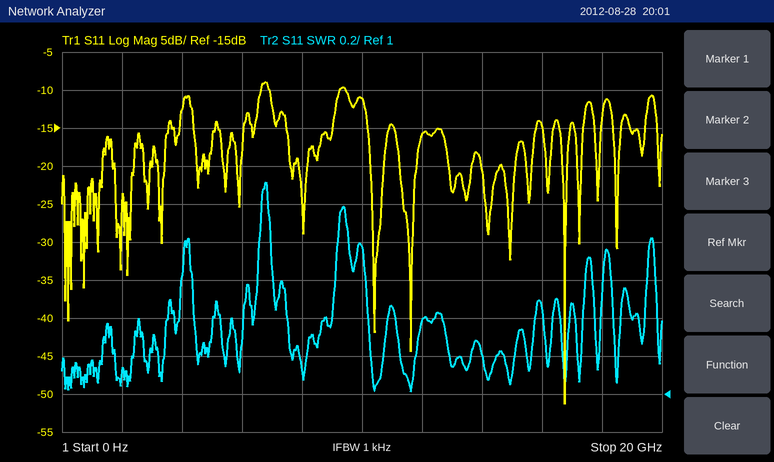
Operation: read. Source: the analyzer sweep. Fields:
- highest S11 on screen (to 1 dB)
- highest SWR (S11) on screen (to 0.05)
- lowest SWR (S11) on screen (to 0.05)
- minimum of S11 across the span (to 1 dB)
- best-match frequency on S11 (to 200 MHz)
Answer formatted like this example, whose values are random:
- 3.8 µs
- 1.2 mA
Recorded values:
- -9 dB
- 2.10
- 1.00
- -51 dB
- 16.8 GHz
